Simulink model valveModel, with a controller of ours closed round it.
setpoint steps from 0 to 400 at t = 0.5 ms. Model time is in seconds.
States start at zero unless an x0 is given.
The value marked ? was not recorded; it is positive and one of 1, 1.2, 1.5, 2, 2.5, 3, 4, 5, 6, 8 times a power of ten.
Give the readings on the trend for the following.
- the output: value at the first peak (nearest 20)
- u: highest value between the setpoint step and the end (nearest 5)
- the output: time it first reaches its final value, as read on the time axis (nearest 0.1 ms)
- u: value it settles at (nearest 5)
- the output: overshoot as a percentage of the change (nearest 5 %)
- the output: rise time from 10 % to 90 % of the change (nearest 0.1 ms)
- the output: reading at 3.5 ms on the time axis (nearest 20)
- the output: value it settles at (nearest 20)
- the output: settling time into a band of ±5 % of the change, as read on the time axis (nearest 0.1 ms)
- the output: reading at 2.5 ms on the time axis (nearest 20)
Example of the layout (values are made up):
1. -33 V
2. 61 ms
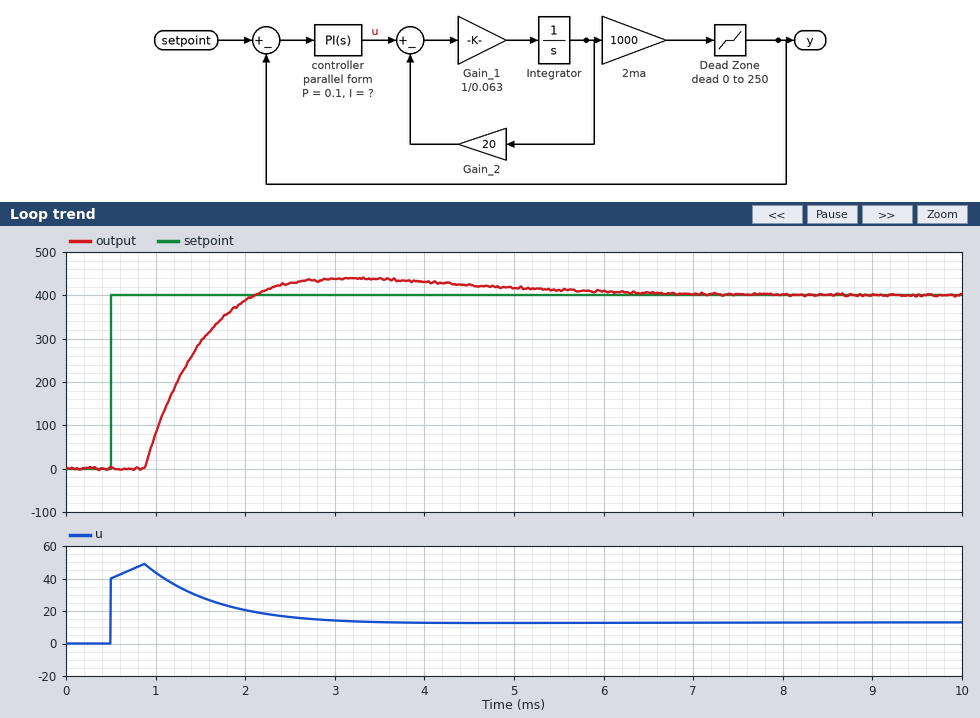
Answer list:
1. 440
2. 50
3. 2.1 ms
4. 15
5. 10 %
6. 0.9 ms
7. 440
8. 400
9. 4.8 ms
10. 420
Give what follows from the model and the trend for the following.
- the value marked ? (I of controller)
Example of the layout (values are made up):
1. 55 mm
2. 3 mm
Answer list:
1. 60
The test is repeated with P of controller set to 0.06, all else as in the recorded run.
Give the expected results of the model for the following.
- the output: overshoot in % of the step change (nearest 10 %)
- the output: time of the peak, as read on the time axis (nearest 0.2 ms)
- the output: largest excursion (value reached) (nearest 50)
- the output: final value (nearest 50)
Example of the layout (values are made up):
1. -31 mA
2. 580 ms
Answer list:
1. 20 %
2. 3.4 ms
3. 500
4. 400
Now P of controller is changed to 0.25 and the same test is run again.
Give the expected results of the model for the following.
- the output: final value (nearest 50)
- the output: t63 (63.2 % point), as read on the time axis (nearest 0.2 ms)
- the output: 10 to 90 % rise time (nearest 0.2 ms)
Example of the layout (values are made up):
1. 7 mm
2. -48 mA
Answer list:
1. 400
2. 1.0 ms
3. 0.6 ms
